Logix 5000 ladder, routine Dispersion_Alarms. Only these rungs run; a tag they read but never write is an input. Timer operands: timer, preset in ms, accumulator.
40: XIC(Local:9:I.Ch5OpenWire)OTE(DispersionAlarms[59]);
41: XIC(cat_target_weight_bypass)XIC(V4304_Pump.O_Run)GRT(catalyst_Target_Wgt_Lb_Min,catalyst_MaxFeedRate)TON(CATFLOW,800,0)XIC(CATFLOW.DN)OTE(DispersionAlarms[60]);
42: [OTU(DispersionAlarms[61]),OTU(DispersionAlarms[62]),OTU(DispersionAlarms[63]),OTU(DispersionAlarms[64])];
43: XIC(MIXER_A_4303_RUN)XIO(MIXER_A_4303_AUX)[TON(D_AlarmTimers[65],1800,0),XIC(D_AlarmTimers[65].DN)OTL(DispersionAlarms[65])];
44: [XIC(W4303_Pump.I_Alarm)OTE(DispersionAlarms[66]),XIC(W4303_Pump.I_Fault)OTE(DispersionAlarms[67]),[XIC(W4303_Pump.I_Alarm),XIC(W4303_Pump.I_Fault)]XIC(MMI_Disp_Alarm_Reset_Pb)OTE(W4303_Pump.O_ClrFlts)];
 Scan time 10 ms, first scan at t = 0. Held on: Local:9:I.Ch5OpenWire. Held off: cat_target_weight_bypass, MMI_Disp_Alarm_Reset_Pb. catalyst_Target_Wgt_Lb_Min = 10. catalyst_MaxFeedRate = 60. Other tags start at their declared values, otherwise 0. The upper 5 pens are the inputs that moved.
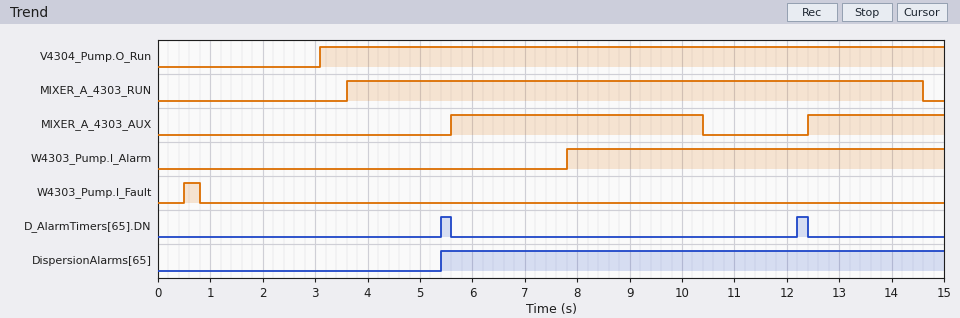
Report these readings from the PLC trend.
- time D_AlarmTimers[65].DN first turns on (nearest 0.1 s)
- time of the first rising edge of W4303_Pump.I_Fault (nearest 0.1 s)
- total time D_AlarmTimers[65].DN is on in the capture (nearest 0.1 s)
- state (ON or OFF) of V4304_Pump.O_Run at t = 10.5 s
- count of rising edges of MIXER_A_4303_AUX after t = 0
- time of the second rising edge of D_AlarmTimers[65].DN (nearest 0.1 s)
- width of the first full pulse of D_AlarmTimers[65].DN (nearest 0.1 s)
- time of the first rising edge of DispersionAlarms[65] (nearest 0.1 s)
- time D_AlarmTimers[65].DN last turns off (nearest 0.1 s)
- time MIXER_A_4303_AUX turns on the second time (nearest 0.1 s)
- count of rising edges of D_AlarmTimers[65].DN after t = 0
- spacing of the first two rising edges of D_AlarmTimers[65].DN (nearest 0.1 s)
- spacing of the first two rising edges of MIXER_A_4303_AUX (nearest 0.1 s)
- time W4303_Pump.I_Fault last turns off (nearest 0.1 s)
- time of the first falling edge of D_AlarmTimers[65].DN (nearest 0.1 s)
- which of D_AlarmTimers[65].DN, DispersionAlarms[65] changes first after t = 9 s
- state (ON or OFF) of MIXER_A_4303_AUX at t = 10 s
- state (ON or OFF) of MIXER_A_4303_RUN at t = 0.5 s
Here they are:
5.4 s
0.5 s
0.4 s
ON
2
12.2 s
0.2 s
5.4 s
12.4 s
12.4 s
2
6.8 s
6.8 s
0.8 s
5.6 s
D_AlarmTimers[65].DN
ON
OFF
